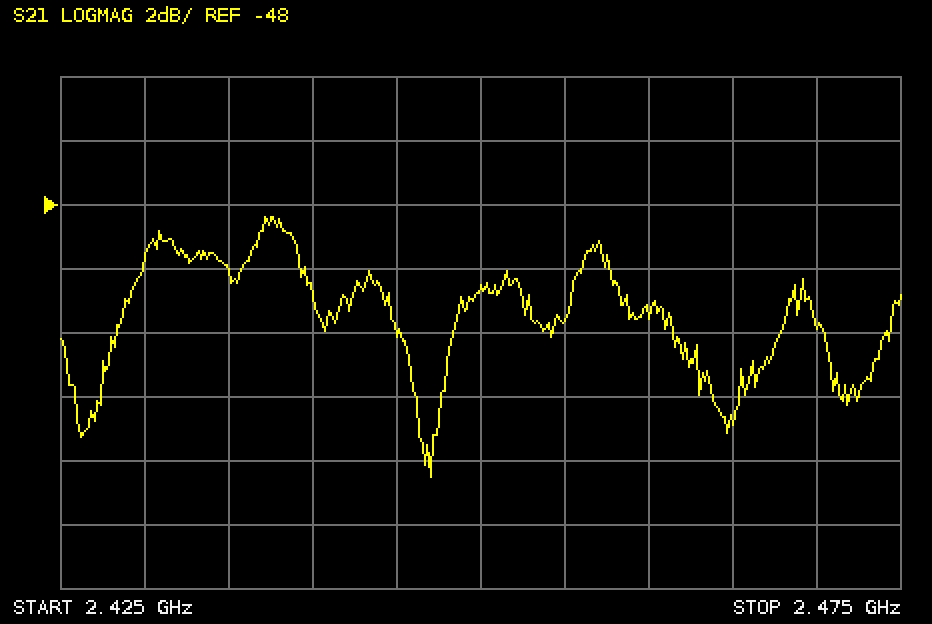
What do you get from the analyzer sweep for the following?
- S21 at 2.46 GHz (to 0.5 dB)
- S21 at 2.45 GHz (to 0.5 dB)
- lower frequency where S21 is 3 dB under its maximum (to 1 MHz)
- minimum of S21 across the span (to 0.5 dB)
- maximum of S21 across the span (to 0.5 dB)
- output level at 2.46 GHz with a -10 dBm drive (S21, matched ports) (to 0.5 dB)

-51.5 dB
-50.5 dB
2.429 GHz
-56.5 dB
-48.5 dB
-61.5 dBm
